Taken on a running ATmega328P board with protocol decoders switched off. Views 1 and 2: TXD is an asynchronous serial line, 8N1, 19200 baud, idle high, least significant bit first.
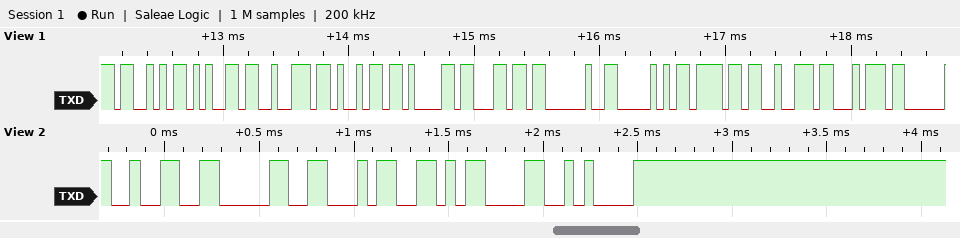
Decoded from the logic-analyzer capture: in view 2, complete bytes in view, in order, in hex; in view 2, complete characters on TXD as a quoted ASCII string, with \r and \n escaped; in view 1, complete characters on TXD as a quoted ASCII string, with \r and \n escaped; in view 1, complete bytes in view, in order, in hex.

0x32 0x30 0x34 0x0D 0x0A
"204\r\n"
"Serial Port"
53 65 72 69 61 6C 20 50 6F 72 74
